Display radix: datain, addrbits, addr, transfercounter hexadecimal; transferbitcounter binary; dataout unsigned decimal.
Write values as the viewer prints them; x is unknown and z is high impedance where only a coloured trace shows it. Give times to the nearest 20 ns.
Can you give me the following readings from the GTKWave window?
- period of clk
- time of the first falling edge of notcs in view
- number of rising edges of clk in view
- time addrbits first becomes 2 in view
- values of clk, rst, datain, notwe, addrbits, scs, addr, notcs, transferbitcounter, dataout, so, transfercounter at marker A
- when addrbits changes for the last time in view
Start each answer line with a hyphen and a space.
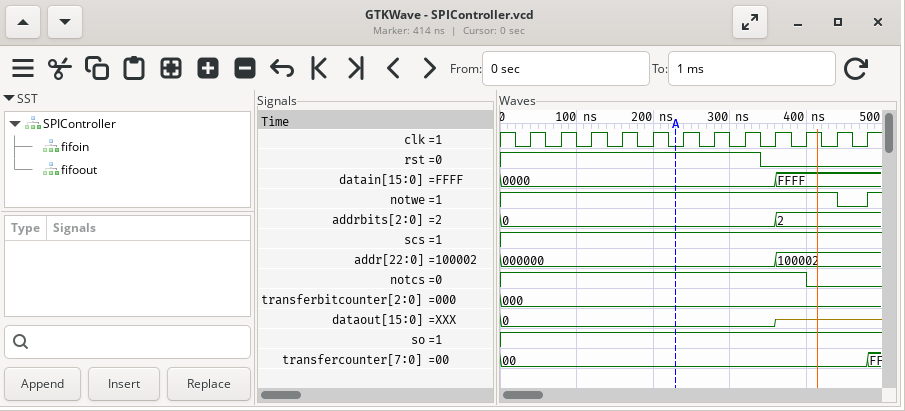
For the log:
- 40 ns
- 400 ns
- 12
- 360 ns
- clk=0, rst=1, datain=0000, notwe=1, addrbits=0, scs=1, addr=000000, notcs=1, transferbitcounter=000, dataout=0, so=1, transfercounter=00
- 360 ns
